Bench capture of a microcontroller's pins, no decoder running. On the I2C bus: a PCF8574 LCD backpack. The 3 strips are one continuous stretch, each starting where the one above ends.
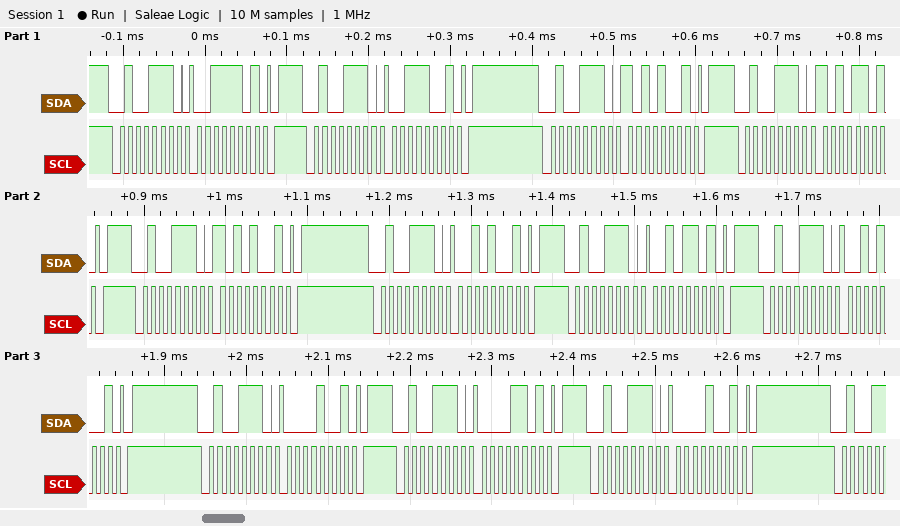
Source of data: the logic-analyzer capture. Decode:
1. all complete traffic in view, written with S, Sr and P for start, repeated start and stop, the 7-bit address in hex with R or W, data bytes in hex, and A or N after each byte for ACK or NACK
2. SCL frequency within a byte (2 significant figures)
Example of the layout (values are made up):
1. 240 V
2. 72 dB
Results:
1. S 27W A 3D A P S 27W A 39 A P S 27W A A9 A P S 27W A AD A P S 27W A A9 A P S 27W A 29 A P S 27W A 2D A P S 27W A 29 A P S 27W A 09 A P S 27W A 0D A P S 27W A 09 A P
2. 100 kHz
